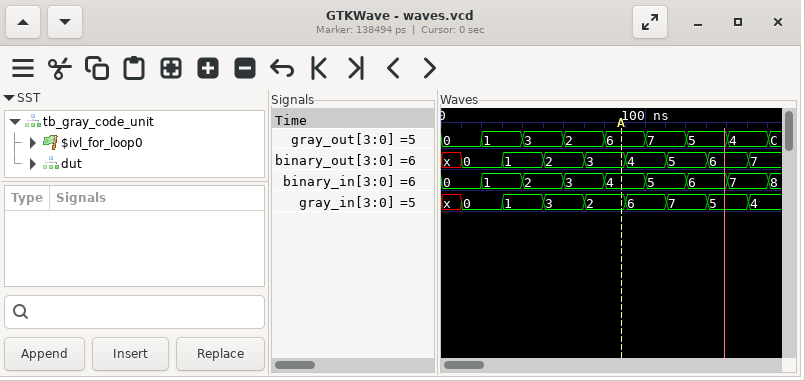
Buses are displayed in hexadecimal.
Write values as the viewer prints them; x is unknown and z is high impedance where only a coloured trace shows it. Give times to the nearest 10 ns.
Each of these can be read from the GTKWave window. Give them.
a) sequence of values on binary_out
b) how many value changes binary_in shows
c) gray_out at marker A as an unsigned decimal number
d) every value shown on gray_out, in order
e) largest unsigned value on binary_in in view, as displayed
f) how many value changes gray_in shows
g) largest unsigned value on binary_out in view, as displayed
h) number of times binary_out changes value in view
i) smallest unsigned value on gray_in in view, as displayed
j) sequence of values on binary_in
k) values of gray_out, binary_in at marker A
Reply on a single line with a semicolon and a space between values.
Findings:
x, 0, 1, 2, 3, 4, 5, 6, 7; 8; 6; 0, 1, 3, 2, 6, 7, 5, 4, C; 8; 8; 7; 8; 0; 0, 1, 2, 3, 4, 5, 6, 7, 8; gray_out=6, binary_in=4
